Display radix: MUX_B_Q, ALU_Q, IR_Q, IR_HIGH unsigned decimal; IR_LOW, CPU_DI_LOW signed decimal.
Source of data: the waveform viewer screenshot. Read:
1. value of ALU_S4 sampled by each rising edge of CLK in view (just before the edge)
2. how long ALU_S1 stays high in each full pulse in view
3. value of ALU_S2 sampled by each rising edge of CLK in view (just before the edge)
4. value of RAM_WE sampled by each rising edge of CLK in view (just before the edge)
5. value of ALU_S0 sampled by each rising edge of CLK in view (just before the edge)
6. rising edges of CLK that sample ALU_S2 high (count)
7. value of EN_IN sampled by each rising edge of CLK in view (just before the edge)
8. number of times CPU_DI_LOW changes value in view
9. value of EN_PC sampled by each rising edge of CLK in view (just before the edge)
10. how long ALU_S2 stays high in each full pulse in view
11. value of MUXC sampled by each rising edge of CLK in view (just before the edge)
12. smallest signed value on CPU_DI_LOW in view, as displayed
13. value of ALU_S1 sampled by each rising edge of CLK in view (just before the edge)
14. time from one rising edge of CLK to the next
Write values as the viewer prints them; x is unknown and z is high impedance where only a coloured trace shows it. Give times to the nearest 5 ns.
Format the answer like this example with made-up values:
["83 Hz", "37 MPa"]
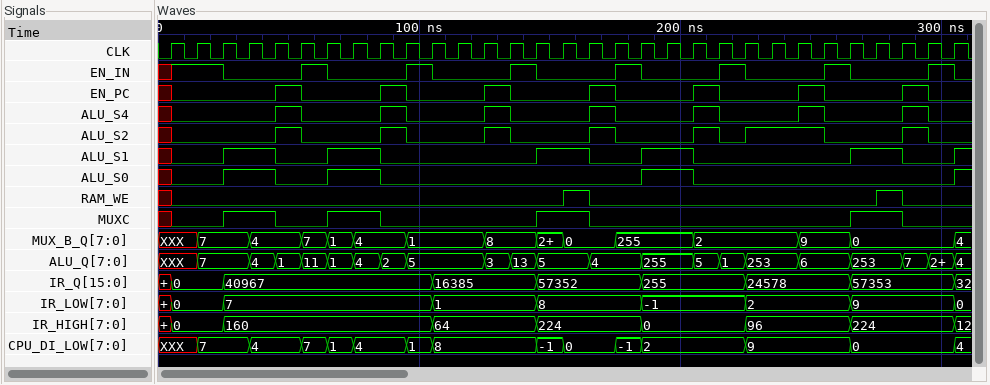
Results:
["x 0 0 0 0 1 0 0 0 1 0 0 0 1 0 0 0 1 0 0 0 1 0 0 0 1 0 0 0 1 0", "20 ns, 20 ns, 20 ns, 20 ns, 20 ns", "x 0 0 0 0 1 0 0 0 1 0 0 0 1 0 0 0 1 0 0 0 1 0 1 1 1 0 0 0 1 0", "x 0 0 0 0 0 0 0 0 0 0 0 0 0 0 0 1 0 0 0 0 0 0 0 0 0 0 0 1 0 0", "x 0 0 1 1 0 0 1 1 0 0 0 0 0 0 0 0 0 0 1 1 0 0 0 0 0 0 0 0 0 0", "9", "x 1 1 0 0 0 1 0 0 0 1 0 0 0 1 0 0 0 1 0 0 0 1 0 0 0 1 0 0 0 1", "14", "x 0 0 0 0 1 0 0 0 1 0 0 0 1 0 0 0 1 0 0 0 1 0 0 0 1 0 0 0 1 0", "10 ns, 10 ns, 10 ns, 10 ns, 10 ns, 30 ns, 10 ns", "x 0 0 1 1 0 0 1 1 0 0 0 0 0 0 1 1 0 0 0 0 0 0 0 0 0 0 1 1 0 0", "-1", "x 0 0 1 1 0 0 1 1 0 0 0 0 0 0 1 1 0 0 1 1 0 0 0 0 0 0 1 1 0 0", "10 ns"]
